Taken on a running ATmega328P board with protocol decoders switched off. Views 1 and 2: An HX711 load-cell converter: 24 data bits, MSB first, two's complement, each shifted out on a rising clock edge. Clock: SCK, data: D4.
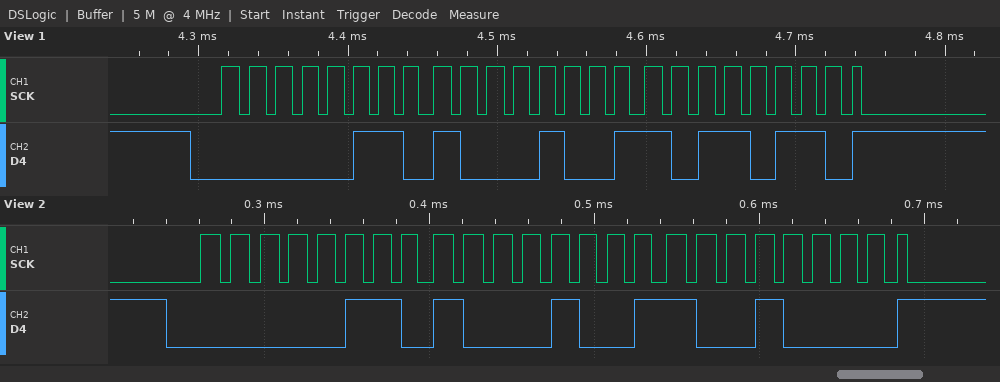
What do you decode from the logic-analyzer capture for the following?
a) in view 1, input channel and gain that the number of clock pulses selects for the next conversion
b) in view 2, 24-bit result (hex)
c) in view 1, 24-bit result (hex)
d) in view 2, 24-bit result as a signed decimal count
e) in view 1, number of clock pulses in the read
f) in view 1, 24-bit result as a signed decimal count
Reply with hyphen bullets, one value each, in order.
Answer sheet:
- channel A, gain 128
- 0x068990
- 0x0689B6
- 428432
- 25
- 428470
